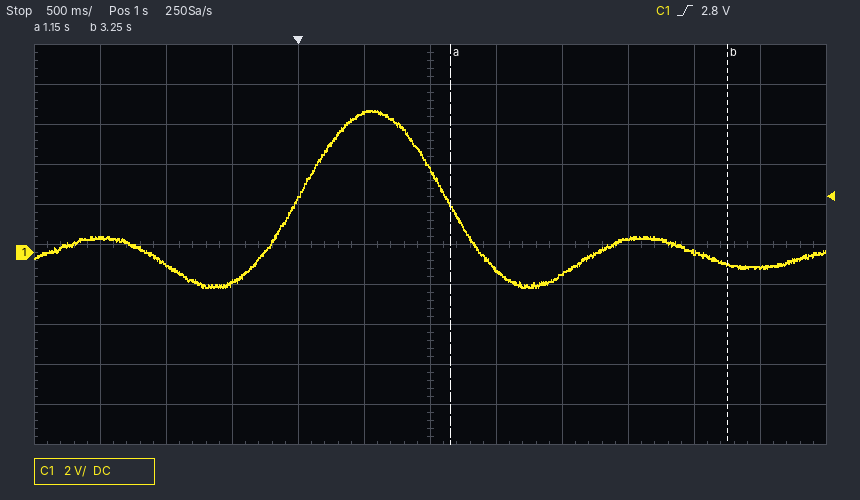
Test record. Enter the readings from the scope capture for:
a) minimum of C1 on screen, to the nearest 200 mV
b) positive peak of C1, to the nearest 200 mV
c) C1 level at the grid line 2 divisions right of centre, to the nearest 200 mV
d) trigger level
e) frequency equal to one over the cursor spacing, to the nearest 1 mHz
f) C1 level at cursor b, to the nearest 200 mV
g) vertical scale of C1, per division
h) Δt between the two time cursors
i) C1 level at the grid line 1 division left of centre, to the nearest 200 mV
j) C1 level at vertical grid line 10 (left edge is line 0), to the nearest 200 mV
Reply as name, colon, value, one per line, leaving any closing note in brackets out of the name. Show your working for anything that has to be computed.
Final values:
minimum of C1 on screen, to the nearest 200 mV: -1.8 V
positive peak of C1, to the nearest 200 mV: 7.2 V
C1 level at the grid line 2 divisions right of centre, to the nearest 200 mV: -1.0 V
trigger level: 2.8 V
frequency equal to one over the cursor spacing, to the nearest 1 mHz: 1 / 2.10 s ≈ 476 mHz
C1 level at cursor b, to the nearest 200 mV: -600 mV
vertical scale of C1, per division: 2 V
Δt between the two time cursors: 3.25 s − (1.15 s) = 2.10 s
C1 level at the grid line 1 division left of centre, to the nearest 200 mV: 7.0 V
C1 level at vertical grid line 10 (left edge is line 0), to the nearest 200 mV: 0.0 V
